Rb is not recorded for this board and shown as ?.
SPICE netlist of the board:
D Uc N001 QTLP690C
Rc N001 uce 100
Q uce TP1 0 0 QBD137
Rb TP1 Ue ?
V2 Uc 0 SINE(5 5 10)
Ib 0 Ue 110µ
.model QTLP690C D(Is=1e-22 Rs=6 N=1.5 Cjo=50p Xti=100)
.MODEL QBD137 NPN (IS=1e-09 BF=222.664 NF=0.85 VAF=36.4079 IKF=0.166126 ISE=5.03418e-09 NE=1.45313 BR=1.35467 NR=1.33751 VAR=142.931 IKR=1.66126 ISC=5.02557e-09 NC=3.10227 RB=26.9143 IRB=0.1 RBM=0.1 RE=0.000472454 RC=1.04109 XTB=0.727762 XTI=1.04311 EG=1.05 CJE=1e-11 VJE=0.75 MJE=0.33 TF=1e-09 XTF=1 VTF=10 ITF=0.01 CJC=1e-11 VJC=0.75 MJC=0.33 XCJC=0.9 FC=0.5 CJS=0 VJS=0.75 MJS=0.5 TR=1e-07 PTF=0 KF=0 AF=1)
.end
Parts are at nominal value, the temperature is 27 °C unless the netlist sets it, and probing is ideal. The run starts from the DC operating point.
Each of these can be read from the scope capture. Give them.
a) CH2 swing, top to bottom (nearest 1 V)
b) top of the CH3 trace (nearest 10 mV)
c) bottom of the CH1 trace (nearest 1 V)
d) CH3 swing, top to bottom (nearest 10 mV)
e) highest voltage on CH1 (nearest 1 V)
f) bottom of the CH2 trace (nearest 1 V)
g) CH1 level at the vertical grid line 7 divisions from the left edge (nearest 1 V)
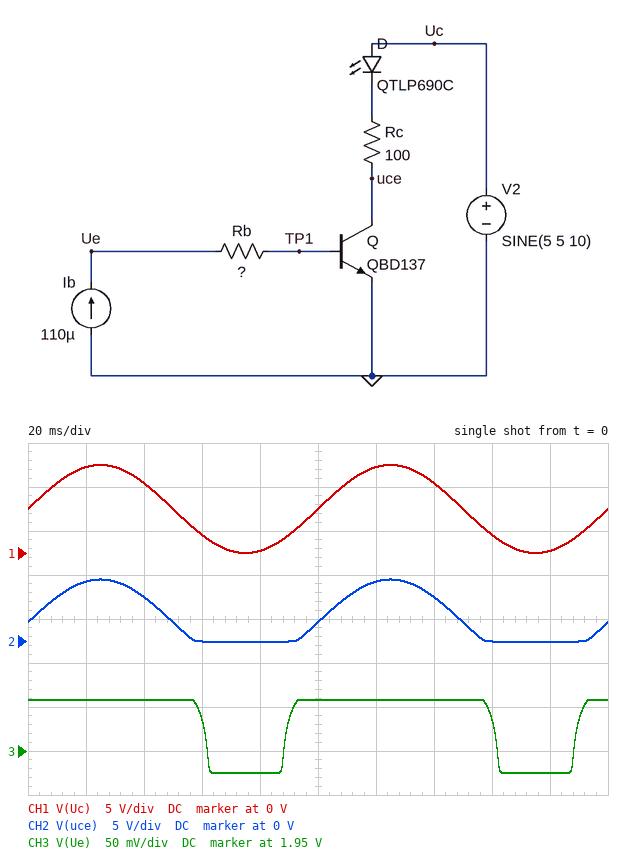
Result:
7 V
2.01 V
0 V
80 mV
10 V
0 V
8 V
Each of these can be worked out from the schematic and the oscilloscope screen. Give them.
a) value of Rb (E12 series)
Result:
15 kΩ
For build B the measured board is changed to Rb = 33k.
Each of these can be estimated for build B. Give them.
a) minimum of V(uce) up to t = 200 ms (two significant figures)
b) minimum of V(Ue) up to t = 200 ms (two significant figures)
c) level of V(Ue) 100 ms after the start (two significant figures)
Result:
-140 mV
3.9 V
4.0 V
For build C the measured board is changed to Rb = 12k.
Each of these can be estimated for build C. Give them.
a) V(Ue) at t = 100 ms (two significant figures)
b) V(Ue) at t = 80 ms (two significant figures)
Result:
1.7 V
1.6 V
